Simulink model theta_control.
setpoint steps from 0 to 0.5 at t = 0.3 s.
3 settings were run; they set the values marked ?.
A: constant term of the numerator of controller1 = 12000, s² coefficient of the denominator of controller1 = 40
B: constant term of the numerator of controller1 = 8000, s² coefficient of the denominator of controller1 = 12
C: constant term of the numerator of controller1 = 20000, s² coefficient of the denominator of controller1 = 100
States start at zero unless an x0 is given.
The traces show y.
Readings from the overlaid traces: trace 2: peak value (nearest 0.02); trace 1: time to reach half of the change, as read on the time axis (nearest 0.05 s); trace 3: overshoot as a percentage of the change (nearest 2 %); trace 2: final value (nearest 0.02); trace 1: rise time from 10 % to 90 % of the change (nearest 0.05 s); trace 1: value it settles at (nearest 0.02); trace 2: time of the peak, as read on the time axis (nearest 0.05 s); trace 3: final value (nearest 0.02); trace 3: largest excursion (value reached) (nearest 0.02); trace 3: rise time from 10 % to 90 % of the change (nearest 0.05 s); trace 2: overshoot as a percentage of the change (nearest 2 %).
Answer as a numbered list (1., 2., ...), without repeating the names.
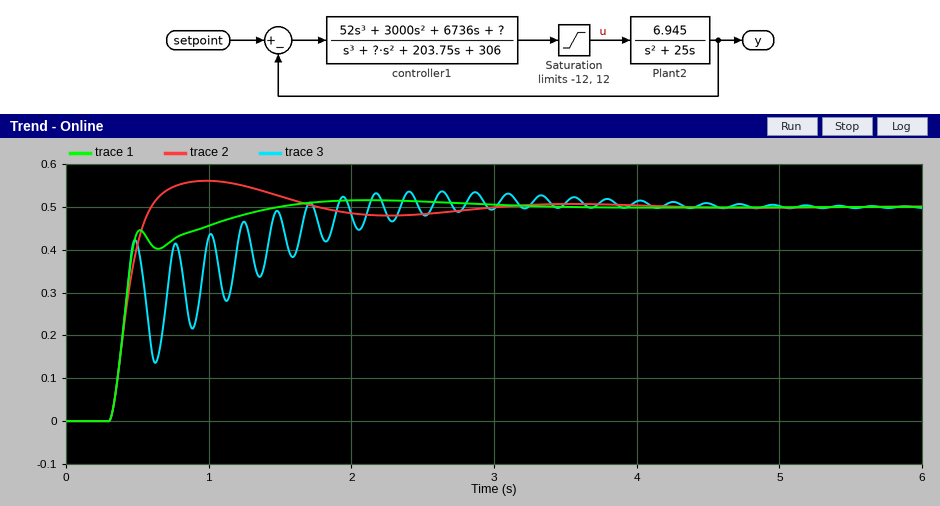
1. 0.56
2. 0.40 s
3. 8 %
4. 0.50
5. 0.60 s
6. 0.50
7. 1.00 s
8. 0.50
9. 0.54
10. 0.90 s
11. 12 %
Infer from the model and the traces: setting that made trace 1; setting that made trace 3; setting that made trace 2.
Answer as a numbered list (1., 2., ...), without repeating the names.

1. A
2. B
3. C
